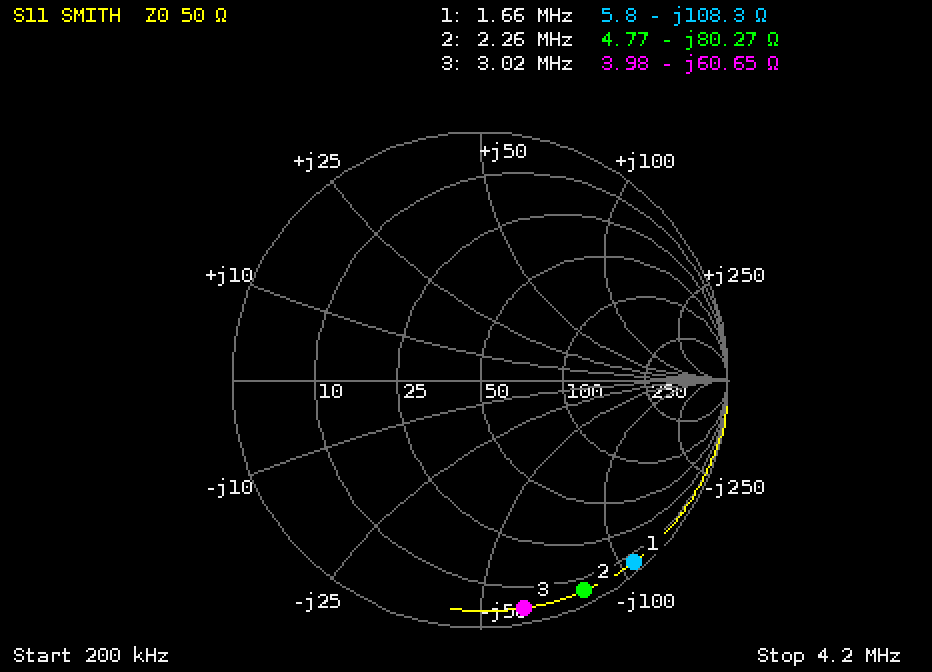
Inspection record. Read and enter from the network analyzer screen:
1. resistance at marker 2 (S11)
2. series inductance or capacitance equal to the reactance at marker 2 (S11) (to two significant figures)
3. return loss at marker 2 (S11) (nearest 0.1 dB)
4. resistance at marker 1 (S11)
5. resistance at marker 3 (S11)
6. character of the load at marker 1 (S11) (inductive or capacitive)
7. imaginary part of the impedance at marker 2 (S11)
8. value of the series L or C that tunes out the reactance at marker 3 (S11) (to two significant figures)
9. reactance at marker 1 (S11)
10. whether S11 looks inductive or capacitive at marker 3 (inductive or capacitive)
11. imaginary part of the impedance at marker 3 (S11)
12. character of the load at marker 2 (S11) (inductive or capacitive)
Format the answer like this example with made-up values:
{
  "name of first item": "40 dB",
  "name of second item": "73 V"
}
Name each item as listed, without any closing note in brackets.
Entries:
{
  "resistance at marker 2": "4.77 Ω",
  "series inductance or capacitance equal to the reactance at marker 2 (S11)": "880 pF",
  "return loss at marker 2 (S11)": "0.5 dB",
  "resistance at marker 1": "5.8 Ω",
  "resistance at marker 3": "3.98 Ω",
  "character of the load at marker 1 (S11)": "capacitive",
  "imaginary part of the impedance at marker 2": "-80.27 Ω",
  "value of the series L or C that tunes out the reactance at marker 3 (S11)": "3.2 µH",
  "reactance at marker 1": "-108.3 Ω",
  "whether S11 looks inductive or capacitive at marker 3": "capacitive",
  "imaginary part of the impedance at marker 3": "-60.65 Ω",
  "character of the load at marker 2 (S11)": "capacitive"
}
